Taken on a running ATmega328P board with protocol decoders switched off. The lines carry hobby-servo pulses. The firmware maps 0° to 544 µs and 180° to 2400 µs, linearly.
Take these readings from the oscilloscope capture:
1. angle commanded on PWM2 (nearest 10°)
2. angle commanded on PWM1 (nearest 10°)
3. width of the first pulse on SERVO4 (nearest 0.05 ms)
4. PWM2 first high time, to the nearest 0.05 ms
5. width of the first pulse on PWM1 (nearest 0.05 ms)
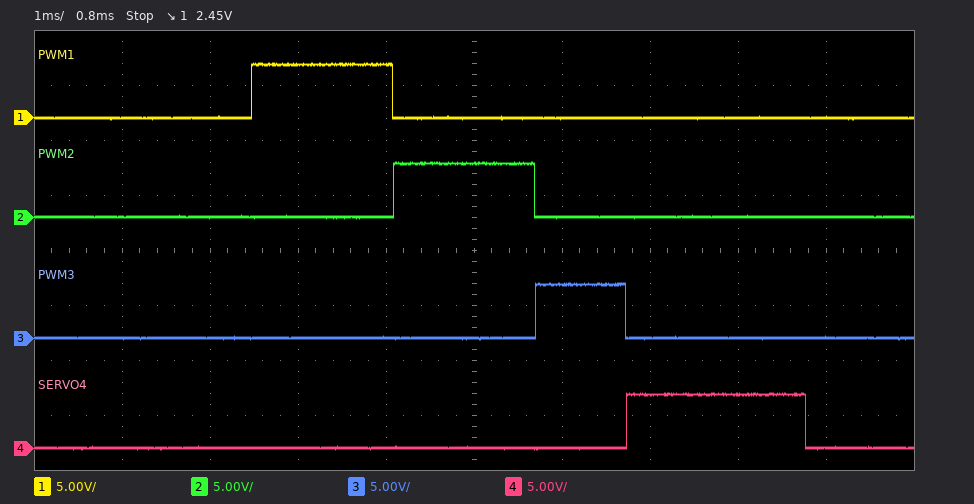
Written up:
100°
100°
2.05 ms
1.60 ms
1.60 ms
